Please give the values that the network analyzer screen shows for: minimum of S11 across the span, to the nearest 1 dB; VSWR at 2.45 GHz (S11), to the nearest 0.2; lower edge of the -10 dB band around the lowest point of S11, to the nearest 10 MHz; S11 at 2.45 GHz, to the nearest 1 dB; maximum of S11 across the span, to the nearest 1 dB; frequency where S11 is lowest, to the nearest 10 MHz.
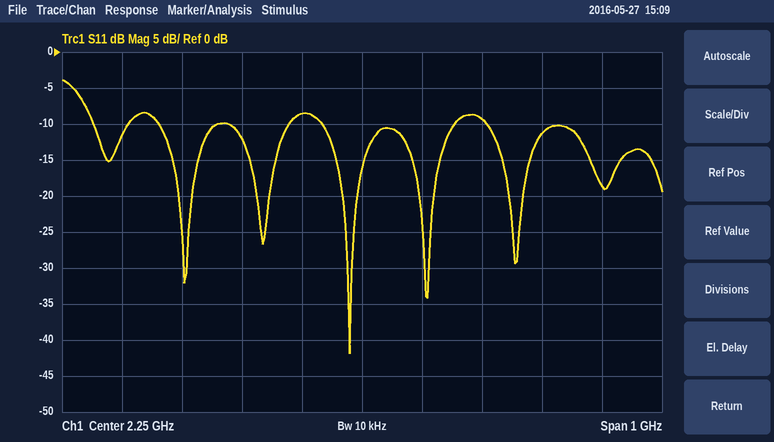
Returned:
-42 dB
2.0
2.18 GHz
-9 dB
-4 dB
2.23 GHz
